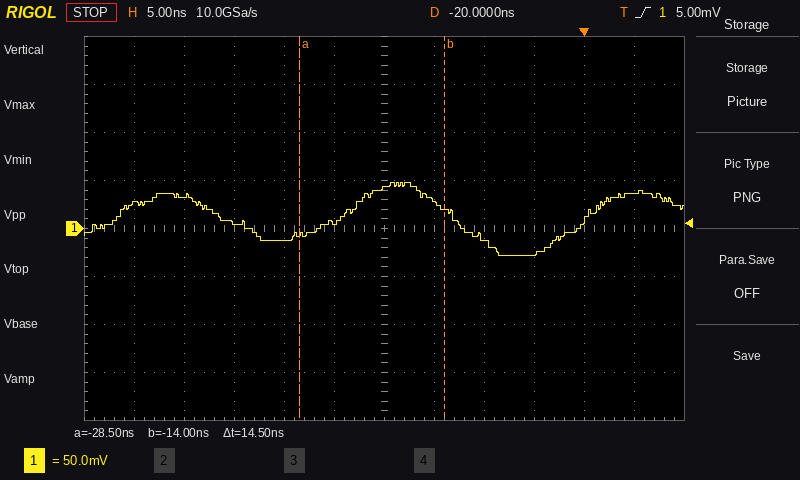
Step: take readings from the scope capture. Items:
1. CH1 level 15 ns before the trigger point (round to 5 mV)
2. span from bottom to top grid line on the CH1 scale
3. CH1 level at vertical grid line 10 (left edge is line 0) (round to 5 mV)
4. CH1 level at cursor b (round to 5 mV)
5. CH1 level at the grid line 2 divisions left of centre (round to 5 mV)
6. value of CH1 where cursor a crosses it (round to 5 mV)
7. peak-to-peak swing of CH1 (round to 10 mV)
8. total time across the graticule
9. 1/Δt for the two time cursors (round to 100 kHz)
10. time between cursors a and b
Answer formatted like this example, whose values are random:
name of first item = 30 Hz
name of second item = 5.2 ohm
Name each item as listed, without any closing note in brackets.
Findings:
CH1 level 15 ns before the trigger point = 30 mV
span from bottom to top grid line on the CH1 scale = 400 mV
CH1 level at vertical grid line 10 (left edge is line 0) = 10 mV
CH1 level at cursor b = 20 mV
CH1 level at the grid line 2 divisions left of centre = -10 mV
value of CH1 where cursor a crosses it = -5 mV
peak-to-peak swing of CH1 = 80 mV
total time across the graticule = 60 ns
1/Δt for the two time cursors = 69.0 MHz
time between cursors a and b = 14.5 ns
